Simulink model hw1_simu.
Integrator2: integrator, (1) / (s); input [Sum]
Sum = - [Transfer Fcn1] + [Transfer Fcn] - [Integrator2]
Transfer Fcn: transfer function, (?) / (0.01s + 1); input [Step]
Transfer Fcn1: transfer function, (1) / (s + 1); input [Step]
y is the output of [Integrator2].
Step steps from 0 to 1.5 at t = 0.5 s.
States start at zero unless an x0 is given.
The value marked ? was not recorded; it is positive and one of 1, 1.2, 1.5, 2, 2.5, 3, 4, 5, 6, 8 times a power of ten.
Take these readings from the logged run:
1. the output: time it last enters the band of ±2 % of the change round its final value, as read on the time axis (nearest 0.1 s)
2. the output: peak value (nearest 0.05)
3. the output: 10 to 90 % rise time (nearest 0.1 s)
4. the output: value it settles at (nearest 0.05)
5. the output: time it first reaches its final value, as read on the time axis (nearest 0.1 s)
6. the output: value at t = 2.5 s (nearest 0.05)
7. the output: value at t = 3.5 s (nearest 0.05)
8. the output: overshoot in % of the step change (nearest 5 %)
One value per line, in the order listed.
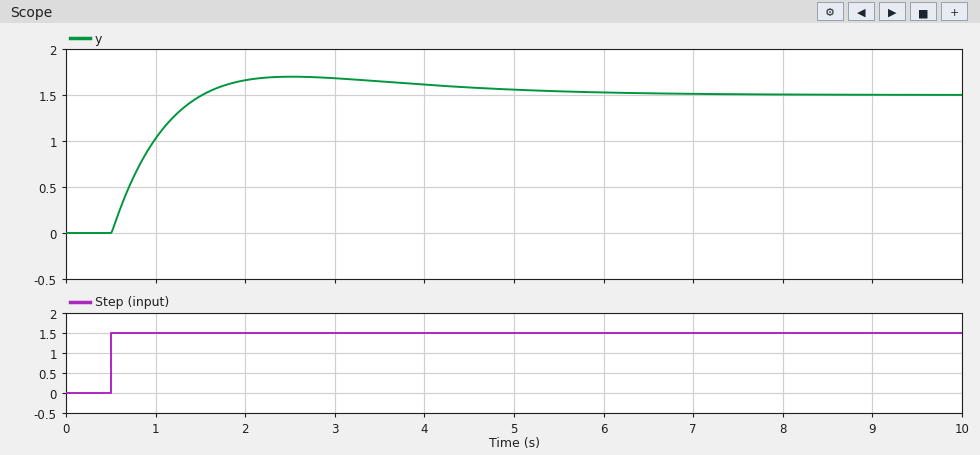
5.9 s
1.70
0.7 s
1.50
1.5 s
1.70
1.65
15 %
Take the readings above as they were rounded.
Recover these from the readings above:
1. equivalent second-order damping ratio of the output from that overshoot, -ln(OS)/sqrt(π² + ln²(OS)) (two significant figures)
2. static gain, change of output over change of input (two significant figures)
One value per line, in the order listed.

0.52
1.0
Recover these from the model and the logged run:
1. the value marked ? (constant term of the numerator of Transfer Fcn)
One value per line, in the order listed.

2
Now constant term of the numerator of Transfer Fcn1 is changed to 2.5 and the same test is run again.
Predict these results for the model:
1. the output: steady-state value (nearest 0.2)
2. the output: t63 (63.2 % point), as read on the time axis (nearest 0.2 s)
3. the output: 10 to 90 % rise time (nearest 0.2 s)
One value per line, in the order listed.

-0.8
4.6 s
2.8 s
